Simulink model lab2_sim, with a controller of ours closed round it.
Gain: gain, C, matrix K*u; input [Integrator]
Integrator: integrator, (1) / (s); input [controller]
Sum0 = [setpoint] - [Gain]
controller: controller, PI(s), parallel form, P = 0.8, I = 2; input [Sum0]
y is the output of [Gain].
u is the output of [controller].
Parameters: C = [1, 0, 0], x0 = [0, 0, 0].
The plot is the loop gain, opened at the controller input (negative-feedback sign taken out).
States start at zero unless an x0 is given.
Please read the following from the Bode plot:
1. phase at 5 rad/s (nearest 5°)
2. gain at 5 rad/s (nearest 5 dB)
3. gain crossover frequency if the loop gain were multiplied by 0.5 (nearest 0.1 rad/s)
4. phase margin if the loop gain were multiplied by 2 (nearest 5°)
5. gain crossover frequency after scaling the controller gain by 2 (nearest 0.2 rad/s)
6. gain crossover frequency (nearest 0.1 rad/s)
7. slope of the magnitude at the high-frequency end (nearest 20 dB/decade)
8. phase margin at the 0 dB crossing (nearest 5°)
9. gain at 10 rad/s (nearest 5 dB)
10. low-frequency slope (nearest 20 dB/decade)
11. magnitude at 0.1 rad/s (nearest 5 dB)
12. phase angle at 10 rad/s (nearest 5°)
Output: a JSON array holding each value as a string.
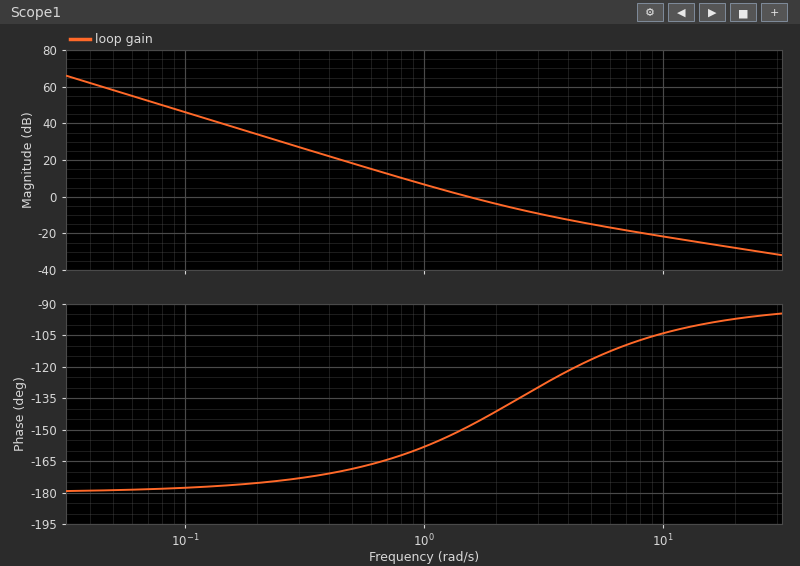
["-115°", "-15 dB", "1.0 rad/s", "45°", "2.4 rad/s", "1.5 rad/s", "-20 dB/decade", "30°", "-20 dB", "-40 dB/decade", "45 dB", "-105°"]
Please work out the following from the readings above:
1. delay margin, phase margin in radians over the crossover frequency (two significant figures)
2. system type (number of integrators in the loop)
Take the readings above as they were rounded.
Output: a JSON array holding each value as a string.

["0.35 s", "2"]
